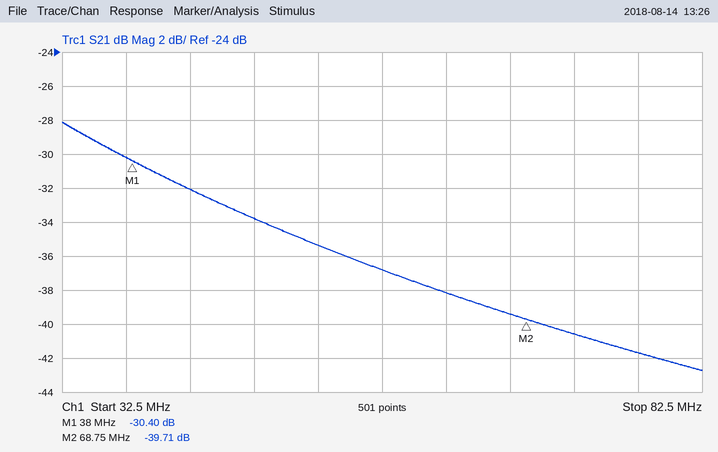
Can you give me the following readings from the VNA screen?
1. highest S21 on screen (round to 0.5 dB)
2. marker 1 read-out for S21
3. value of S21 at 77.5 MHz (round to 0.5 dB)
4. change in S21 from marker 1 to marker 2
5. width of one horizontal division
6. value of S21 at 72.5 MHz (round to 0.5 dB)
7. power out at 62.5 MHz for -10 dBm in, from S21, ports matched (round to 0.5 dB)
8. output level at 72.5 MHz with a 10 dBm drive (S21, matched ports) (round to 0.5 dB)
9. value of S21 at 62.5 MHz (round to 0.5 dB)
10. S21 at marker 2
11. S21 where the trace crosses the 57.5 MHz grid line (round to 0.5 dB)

-28.0 dB
-30.40 dB
-41.5 dB
-9.31 dB
5 MHz
-40.5 dB
-48.0 dBm
-30.5 dBm
-38.0 dB
-39.71 dB
-37.0 dB
